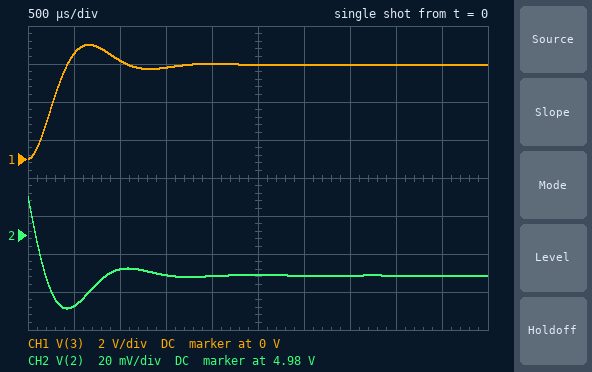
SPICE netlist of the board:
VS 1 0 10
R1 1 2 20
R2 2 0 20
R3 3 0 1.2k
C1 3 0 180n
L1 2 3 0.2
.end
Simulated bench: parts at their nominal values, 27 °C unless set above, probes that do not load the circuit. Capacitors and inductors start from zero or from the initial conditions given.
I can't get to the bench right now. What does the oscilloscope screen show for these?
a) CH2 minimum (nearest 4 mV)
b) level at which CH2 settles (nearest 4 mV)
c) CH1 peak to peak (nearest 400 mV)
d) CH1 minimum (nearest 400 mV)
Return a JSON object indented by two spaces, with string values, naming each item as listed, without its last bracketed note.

{
  "CH2 minimum": "4.940 V",
  "level at which CH2 settles": "4.960 V",
  "CH1 peak to peak": "6.0 V",
  "CH1 minimum": "0 V"
}
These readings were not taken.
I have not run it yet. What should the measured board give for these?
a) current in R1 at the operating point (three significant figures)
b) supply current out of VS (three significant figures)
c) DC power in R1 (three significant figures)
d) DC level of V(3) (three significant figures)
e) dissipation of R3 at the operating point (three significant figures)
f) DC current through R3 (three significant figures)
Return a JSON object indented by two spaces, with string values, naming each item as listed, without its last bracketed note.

{
  "current in R1 at the operating point": "252 mA",
  "supply current out of VS": "252 mA",
  "DC power in R1": "1.27 W",
  "DC level of V(3)": "4.96 V",
  "dissipation of R3 at the operating point": "20.5 mW",
  "DC current through R3": "4.13 mA"
}
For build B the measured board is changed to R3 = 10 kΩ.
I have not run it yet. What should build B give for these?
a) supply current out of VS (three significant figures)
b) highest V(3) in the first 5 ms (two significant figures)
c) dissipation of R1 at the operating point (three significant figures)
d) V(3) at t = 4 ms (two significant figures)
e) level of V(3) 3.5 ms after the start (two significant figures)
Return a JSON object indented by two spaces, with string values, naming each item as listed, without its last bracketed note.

{
  "supply current out of VS": "250 mA",
  "highest V(3) in the first 5 ms": "9.2 V",
  "dissipation of R1 at the operating point": "1.25 W",
  "V(3) at t = 4 ms": "5.8 V",
  "level of V(3) 3.5 ms after the start": "3.5 V"
}
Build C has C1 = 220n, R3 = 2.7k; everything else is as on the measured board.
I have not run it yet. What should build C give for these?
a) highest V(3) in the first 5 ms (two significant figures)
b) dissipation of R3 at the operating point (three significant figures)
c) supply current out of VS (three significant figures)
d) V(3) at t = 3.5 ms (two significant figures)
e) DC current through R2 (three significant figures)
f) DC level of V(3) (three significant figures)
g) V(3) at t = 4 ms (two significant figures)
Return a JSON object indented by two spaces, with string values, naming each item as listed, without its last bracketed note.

{
  "highest V(3) in the first 5 ms": "7.8 V",
  "dissipation of R3 at the operating point": "9.19 mW",
  "supply current out of VS": "251 mA",
  "V(3) at t = 3.5 ms": "5.2 V",
  "DC current through R2": "249 mA",
  "DC level of V(3)": "4.98 V",
  "V(3) at t = 4 ms": "4.8 V"
}
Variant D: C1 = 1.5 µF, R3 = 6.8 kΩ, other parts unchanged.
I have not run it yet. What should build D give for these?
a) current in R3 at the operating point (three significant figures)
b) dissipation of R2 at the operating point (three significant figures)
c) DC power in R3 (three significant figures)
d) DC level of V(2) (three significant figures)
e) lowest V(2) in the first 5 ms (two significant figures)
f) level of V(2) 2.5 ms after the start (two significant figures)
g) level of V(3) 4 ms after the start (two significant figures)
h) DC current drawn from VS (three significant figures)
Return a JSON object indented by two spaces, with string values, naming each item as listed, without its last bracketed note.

{
  "current in R3 at the operating point": "734 µA",
  "dissipation of R2 at the operating point": "1.25 W",
  "DC power in R3": "3.67 mW",
  "DC level of V(2)": "4.99 V",
  "lowest V(2) in the first 5 ms": "4.9 V",
  "level of V(2) 2.5 ms after the start": "5.1 V",
  "level of V(3) 4 ms after the start": "2.9 V",
  "DC current drawn from VS": "250 mA"
}
